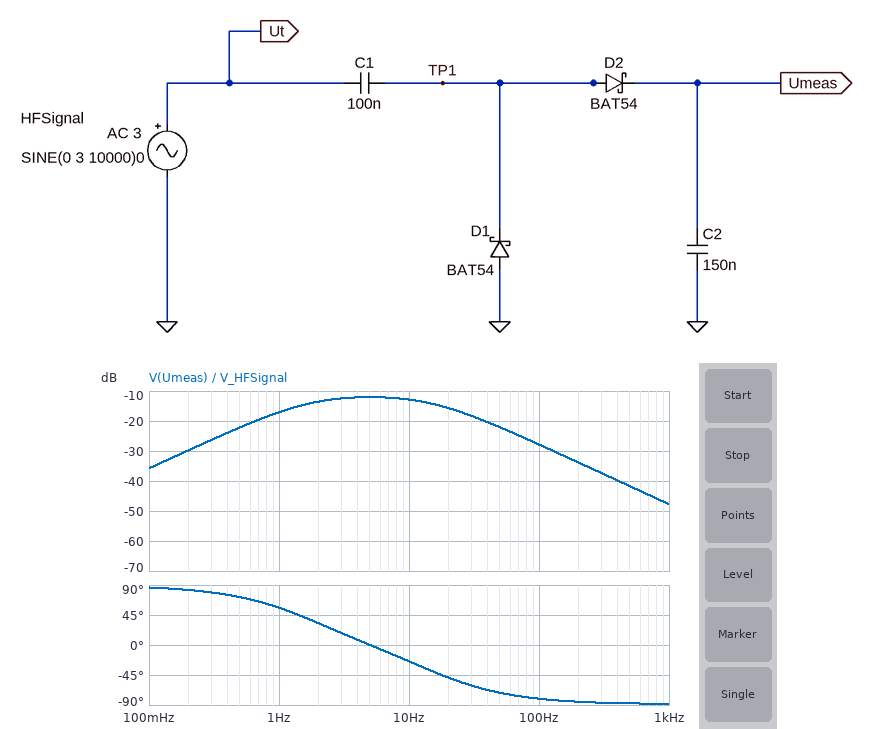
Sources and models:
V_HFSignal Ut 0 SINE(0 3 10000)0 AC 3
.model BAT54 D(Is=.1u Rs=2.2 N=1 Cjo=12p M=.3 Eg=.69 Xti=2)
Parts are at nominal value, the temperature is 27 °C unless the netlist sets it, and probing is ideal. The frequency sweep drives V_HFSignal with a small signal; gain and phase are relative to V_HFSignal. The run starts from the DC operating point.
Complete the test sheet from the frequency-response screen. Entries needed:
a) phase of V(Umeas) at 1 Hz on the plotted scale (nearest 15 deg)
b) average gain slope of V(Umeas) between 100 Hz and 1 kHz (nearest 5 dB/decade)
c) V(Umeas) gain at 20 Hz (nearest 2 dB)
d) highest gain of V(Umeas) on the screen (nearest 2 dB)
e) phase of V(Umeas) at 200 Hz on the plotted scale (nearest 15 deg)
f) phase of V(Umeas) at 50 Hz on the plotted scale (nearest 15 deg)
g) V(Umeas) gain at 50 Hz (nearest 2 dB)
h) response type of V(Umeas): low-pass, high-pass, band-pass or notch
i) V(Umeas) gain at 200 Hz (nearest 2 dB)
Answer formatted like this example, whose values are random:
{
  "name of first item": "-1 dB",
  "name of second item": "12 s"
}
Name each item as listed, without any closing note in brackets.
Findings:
{
  "phase of V(Umeas) at 1 Hz on the plotted scale": "60 deg",
  "average gain slope of V(Umeas) between 100 Hz and 1 kHz": "-20 dB/decade",
  "V(Umeas) gain at 20 Hz": "-16 dB",
  "highest gain of V(Umeas) on the screen": "-12 dB",
  "phase of V(Umeas) at 200 Hz on the plotted scale": "-90 deg",
  "phase of V(Umeas) at 50 Hz on the plotted scale": "-75 deg",
  "V(Umeas) gain at 50 Hz": "-22 dB",
  "response type of V(Umeas): low-pass, high-pass, band-pass or notch": "band-pass",
  "V(Umeas) gain at 200 Hz": "-34 dB"
}
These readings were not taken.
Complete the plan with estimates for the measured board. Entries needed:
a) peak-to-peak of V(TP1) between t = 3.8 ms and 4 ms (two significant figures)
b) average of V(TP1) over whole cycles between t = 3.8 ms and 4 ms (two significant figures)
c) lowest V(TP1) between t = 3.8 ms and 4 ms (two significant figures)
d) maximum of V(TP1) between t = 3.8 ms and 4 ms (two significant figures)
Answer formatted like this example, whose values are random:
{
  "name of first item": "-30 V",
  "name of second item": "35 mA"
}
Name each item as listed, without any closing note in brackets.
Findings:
{
  "peak-to-peak of V(TP1) between t = 3.8 ms and 4 ms": "6.0 V",
  "average of V(TP1) over whole cycles between t = 3.8 ms and 4 ms": "2.8 V",
  "lowest V(TP1) between t = 3.8 ms and 4 ms": "-180 mV",
  "maximum of V(TP1) between t = 3.8 ms and 4 ms": "5.8 V"
}
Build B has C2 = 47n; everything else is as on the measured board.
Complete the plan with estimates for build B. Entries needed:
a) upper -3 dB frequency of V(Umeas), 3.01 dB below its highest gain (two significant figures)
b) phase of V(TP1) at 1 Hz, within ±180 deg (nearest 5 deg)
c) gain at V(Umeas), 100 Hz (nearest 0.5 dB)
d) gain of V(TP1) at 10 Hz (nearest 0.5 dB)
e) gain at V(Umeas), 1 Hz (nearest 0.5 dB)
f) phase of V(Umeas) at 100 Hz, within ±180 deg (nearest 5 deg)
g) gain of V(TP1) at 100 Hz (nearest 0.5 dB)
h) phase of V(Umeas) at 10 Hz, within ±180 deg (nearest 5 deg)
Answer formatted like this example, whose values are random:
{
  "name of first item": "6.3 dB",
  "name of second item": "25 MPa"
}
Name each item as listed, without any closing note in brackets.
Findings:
{
  "upper -3 dB frequency of V(Umeas), 3.01 dB below its highest gain": "28 Hz",
  "phase of V(TP1) at 1 Hz, within ±180 deg": "75 deg",
  "gain at V(Umeas), 100 Hz": "-18.0 dB",
  "gain of V(TP1) at 10 Hz": "-4.0 dB",
  "gain at V(Umeas), 1 Hz": "-16.0 dB",
  "phase of V(Umeas) at 100 Hz, within ±180 deg": "-75 deg",
  "gain of V(TP1) at 100 Hz": "0 dB",
  "phase of V(Umeas) at 10 Hz, within ±180 deg": "-5 deg"
}
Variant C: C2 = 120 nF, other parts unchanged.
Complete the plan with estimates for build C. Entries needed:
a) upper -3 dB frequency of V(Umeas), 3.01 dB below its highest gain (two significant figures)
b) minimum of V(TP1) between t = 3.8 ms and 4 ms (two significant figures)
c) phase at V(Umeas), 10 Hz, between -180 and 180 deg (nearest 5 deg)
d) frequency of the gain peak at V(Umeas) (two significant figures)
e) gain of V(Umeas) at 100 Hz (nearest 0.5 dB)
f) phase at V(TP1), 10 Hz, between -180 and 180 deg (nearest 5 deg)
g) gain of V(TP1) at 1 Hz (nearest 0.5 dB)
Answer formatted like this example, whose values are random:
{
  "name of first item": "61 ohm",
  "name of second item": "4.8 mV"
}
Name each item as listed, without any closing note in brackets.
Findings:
{
  "upper -3 dB frequency of V(Umeas), 3.01 dB below its highest gain": "19 Hz",
  "minimum of V(TP1) between t = 3.8 ms and 4 ms": "-170 mV",
  "phase at V(Umeas), 10 Hz, between -180 and 180 deg": "-20 deg",
  "frequency of the gain peak at V(Umeas)": "5.6 Hz",
  "gain of V(Umeas) at 100 Hz": "-26.0 dB",
  "phase at V(TP1), 10 Hz, between -180 and 180 deg": "40 deg",
  "gain of V(TP1) at 1 Hz": "-16.5 dB"
}
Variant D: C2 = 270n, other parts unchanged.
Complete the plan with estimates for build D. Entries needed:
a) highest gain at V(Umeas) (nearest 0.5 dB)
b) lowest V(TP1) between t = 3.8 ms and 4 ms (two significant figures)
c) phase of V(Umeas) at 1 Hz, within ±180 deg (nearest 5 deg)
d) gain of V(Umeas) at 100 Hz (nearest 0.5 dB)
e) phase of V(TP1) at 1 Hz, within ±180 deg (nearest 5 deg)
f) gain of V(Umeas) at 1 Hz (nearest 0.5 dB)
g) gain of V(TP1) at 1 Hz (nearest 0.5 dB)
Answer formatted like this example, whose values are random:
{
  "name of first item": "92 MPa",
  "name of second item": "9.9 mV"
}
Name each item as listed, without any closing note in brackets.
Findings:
{
  "highest gain at V(Umeas)": "-16.0 dB",
  "lowest V(TP1) between t = 3.8 ms and 4 ms": "-190 mV",
  "phase of V(Umeas) at 1 Hz, within ±180 deg": "40 deg",
  "gain of V(Umeas) at 100 Hz": "-33.0 dB",
  "phase of V(TP1) at 1 Hz, within ±180 deg": "65 deg",
  "gain of V(Umeas) at 1 Hz": "-18.5 dB",
  "gain of V(TP1) at 1 Hz": "-18.0 dB"
}
